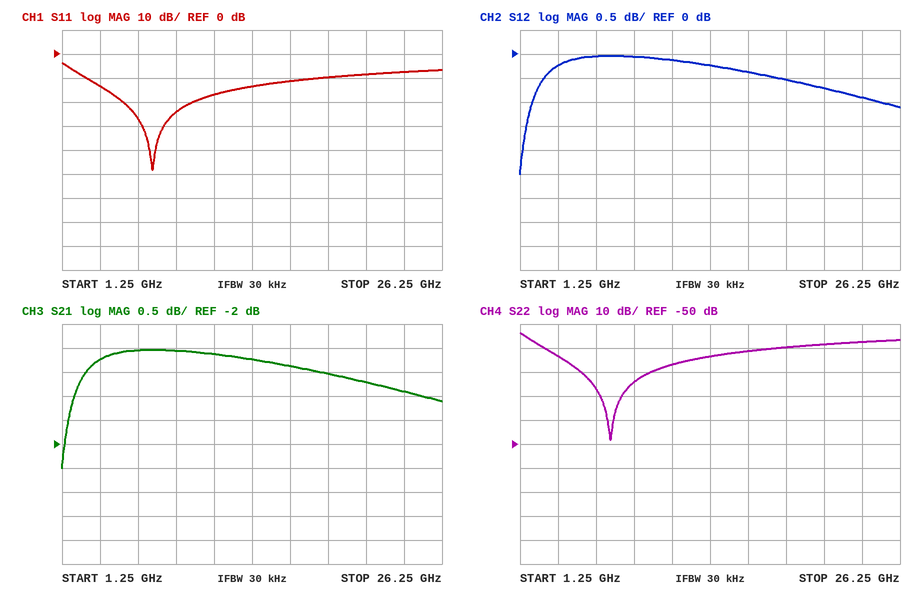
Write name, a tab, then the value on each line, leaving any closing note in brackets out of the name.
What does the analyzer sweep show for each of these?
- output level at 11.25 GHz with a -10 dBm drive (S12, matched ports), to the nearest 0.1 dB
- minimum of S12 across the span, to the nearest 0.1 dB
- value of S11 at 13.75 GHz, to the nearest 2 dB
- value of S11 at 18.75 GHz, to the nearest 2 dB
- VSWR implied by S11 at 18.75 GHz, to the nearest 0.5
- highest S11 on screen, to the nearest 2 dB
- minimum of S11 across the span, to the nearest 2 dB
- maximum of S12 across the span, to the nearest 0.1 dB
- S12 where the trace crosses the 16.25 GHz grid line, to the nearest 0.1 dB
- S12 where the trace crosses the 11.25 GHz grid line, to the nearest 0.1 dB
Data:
output level at 11.25 GHz with a -10 dBm drive (S12, matched ports), to the nearest 0.1 dB	-10.1 dBm
minimum of S12 across the span, to the nearest 0.1 dB	-2.5 dB
value of S11 at 13.75 GHz, to the nearest 2 dB	-14 dB
value of S11 at 18.75 GHz, to the nearest 2 dB	-10 dB
VSWR implied by S11 at 18.75 GHz, to the nearest 0.5	2.0
highest S11 on screen, to the nearest 2 dB	-4 dB
minimum of S11 across the span, to the nearest 2 dB	-48 dB
maximum of S12 across the span, to the nearest 0.1 dB	0.0 dB
S12 where the trace crosses the 16.25 GHz grid line, to the nearest 0.1 dB	-0.4 dB
S12 where the trace crosses the 11.25 GHz grid line, to the nearest 0.1 dB	-0.1 dB
